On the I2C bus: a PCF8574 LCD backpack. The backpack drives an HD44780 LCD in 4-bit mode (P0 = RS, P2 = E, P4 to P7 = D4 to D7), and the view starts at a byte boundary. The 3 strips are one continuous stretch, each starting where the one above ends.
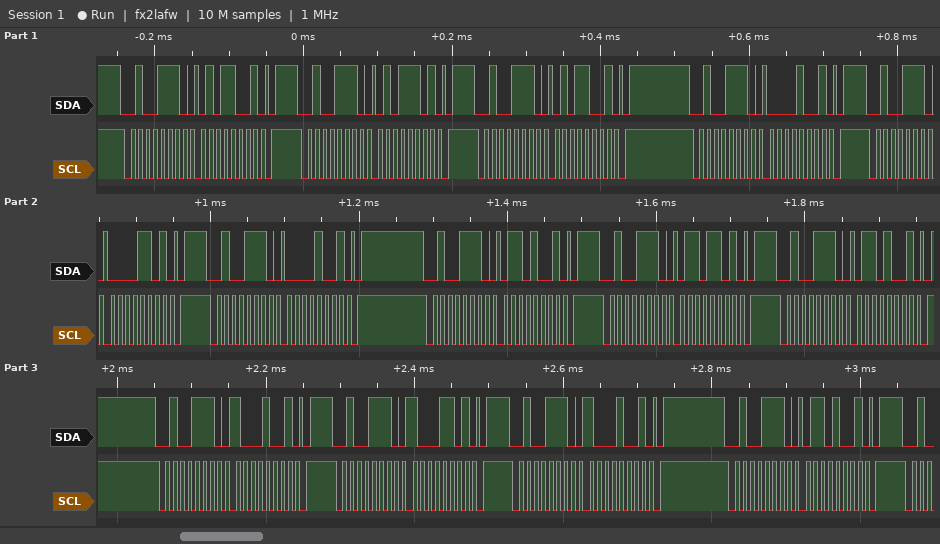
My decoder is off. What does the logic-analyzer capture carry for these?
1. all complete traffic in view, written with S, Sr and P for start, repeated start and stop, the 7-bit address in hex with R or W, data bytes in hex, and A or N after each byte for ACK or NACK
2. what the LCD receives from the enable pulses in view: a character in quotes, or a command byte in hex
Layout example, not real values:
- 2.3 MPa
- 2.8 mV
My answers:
- S 27W A 59 A P S 27W A 5D A P S 27W A 59 A P S 27W A 09 A P S 27W A 0D A P S 27W A 09 A P S 27W A 69 A P S 27W A 6D A P S 27W A 69 A P S 27W A 89 A P S 27W A 8D A P S 27W A 89 A P S 27W A 69 A P
- 'P' 'h'
